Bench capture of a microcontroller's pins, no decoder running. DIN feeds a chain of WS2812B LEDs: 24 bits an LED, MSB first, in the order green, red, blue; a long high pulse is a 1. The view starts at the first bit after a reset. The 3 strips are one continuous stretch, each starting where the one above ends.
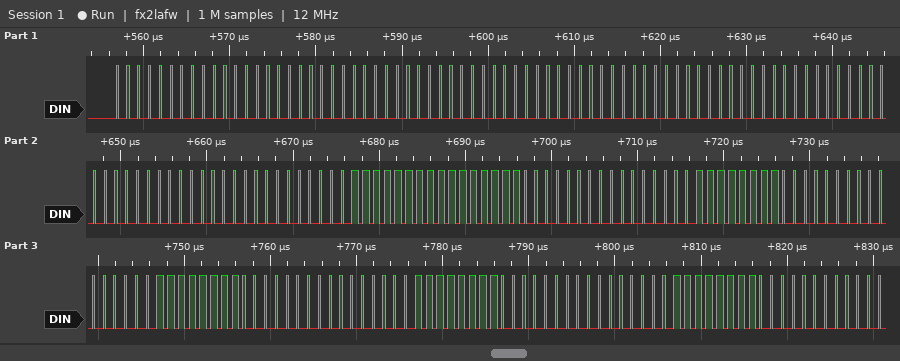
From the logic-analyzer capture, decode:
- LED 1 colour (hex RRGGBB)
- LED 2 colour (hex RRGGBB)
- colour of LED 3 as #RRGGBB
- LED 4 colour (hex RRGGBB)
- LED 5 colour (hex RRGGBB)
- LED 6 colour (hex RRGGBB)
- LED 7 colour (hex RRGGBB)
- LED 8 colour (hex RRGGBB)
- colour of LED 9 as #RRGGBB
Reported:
#000000
#000000
#000000
#000000
#FFFF00
#FF0000
#FF0000
#FF0000
#FF0000
